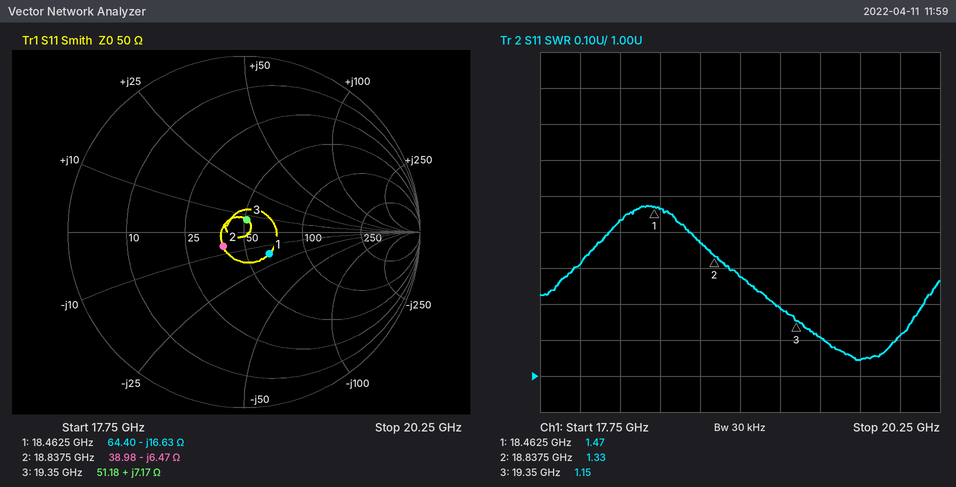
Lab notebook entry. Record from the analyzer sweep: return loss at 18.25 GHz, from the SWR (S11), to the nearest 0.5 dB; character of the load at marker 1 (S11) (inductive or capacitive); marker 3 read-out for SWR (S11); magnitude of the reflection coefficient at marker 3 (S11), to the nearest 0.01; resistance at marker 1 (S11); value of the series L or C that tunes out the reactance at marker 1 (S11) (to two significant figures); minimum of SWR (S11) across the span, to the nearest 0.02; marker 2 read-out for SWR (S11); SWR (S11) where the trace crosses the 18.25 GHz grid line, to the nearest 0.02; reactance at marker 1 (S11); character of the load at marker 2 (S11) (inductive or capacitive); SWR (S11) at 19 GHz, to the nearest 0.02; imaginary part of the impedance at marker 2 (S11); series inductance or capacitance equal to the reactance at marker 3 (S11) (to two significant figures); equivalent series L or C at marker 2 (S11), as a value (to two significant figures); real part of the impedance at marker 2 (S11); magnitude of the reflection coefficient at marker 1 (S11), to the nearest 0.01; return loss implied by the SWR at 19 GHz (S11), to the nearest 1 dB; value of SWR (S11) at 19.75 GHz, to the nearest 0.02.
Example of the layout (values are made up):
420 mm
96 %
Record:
15.0 dB
capacitive
1.15
0.07
64.40 Ω
140 pH
1.04
1.33
1.44
-16.63 Ω
capacitive
1.28
-6.47 Ω
59 pH
1.3 pF
38.98 Ω
0.19
18 dB
1.04
